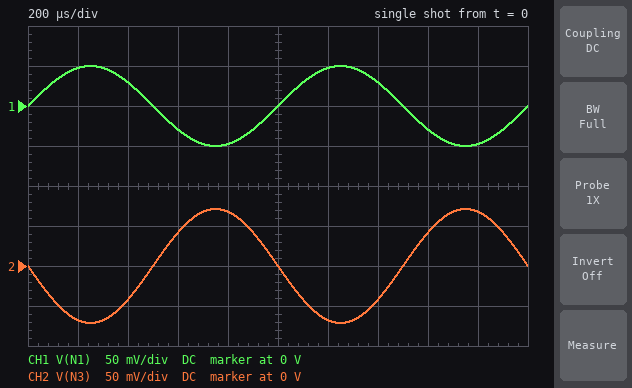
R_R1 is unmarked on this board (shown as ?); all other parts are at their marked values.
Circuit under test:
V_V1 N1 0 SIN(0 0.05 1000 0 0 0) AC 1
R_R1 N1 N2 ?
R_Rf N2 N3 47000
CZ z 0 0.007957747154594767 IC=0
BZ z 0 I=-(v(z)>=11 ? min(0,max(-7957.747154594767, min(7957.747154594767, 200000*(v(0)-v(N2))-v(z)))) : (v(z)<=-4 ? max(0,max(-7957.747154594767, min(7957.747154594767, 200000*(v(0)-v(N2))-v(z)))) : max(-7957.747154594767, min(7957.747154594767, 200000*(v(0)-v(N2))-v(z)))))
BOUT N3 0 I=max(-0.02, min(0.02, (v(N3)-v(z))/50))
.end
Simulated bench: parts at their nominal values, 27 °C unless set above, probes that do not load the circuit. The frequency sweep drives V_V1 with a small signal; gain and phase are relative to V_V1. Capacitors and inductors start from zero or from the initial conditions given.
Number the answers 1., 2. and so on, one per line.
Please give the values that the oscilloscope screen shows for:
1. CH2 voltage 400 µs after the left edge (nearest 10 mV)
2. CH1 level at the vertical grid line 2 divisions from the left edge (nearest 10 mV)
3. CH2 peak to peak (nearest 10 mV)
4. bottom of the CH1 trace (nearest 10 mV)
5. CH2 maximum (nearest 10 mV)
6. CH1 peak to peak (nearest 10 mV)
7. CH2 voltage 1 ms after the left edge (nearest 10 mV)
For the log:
1. -40 mV
2. 30 mV
3. 140 mV
4. -50 mV
5. 70 mV
6. 100 mV
7. 0 V
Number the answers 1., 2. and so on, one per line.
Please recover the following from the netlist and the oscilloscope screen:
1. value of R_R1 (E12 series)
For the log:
1. 33 kΩ
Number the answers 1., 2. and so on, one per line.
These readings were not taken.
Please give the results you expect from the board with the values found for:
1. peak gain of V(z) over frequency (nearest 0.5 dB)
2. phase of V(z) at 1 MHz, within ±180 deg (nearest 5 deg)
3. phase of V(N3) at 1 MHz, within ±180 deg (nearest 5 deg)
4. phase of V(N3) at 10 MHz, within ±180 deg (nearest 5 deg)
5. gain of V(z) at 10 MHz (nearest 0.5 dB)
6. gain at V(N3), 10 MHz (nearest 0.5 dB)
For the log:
1. 3.0 dB
2. 150 deg
3. 150 deg
4. 100 deg
5. -12.5 dB
6. -12.5 dB
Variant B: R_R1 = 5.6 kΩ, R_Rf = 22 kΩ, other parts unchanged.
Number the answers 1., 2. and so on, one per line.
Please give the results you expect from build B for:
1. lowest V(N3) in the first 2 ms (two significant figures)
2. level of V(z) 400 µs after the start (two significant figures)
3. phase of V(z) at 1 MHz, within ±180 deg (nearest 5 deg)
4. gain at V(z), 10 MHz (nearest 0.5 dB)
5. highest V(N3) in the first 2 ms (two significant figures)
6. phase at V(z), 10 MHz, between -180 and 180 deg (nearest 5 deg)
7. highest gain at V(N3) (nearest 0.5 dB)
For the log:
1. -200 mV
2. -120 mV
3. 130 deg
4. -10.0 dB
5. 200 mV
6. 95 deg
7. 12.0 dB
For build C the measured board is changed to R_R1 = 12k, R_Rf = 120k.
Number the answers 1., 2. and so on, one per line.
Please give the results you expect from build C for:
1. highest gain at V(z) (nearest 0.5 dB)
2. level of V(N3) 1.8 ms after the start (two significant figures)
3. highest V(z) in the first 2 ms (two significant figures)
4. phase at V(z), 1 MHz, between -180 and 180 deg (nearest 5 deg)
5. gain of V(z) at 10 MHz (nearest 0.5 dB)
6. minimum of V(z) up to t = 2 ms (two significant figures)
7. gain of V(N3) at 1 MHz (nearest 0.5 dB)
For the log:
1. 20.0 dB
2. 480 mV
3. 500 mV
4. 110 deg
5. -9.0 dB
6. -500 mV
7. 10.5 dB
